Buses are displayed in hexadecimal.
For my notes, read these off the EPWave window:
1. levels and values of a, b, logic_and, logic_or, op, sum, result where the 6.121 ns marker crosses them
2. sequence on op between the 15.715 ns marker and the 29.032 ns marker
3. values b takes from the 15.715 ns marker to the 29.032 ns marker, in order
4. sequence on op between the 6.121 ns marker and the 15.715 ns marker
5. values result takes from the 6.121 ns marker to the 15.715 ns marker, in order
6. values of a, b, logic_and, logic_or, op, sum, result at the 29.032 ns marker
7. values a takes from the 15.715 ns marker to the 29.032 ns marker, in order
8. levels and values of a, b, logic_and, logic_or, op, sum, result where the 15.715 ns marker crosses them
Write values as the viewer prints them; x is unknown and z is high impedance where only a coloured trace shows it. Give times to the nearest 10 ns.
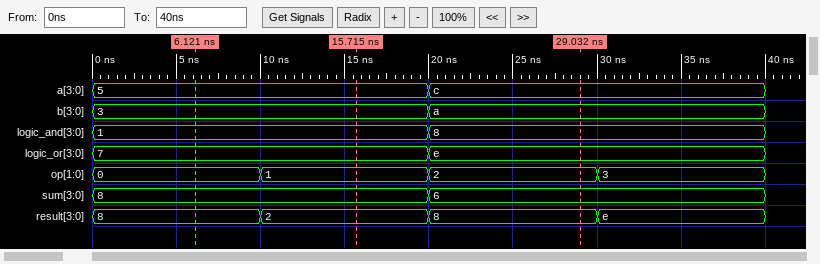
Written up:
a=5, b=3, logic_and=1, logic_or=7, op=0, sum=8, result=8
1, 2
3, a
0, 1
8, 2
a=c, b=a, logic_and=8, logic_or=e, op=2, sum=6, result=8
5, c
a=5, b=3, logic_and=1, logic_or=7, op=1, sum=8, result=2
